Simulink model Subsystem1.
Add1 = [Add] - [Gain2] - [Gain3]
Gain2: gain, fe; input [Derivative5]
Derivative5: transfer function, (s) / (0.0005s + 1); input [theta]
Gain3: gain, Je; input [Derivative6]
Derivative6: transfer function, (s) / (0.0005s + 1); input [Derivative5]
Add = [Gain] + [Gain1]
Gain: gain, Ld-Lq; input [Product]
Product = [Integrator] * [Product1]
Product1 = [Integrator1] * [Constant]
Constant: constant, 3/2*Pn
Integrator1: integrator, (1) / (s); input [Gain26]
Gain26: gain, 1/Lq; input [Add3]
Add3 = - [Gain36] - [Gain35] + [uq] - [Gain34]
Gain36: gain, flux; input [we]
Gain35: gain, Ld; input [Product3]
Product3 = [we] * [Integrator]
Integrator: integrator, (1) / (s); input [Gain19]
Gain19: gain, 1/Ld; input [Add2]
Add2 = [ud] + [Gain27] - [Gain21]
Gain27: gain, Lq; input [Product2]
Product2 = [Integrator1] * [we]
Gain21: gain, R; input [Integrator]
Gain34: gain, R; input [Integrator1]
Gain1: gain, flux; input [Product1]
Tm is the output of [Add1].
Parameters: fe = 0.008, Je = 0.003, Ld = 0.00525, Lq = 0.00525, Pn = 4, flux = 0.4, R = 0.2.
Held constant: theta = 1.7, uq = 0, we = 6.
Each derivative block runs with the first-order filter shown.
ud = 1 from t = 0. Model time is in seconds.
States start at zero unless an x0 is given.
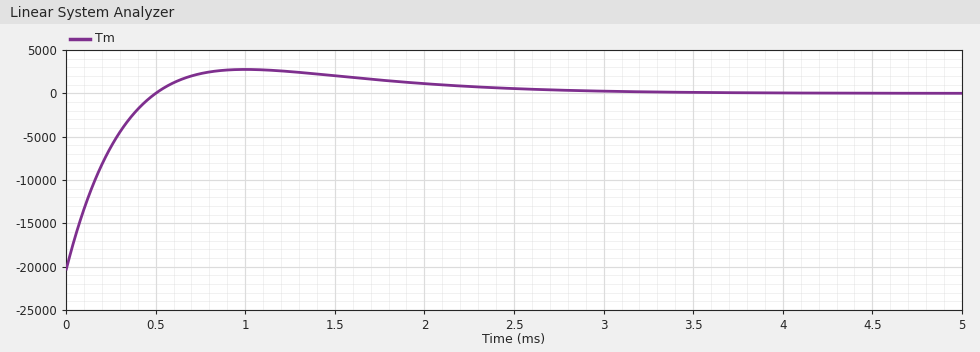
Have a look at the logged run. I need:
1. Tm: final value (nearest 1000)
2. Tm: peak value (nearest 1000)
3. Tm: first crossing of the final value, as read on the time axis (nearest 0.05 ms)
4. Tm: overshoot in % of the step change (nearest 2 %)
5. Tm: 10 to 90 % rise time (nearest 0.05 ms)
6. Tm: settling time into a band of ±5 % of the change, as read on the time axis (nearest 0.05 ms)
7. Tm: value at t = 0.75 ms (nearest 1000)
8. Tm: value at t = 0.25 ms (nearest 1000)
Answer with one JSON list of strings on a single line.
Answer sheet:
["0", "3000", "0.50 ms", "14 %", "0.35 ms", "2.10 ms", "2000", "-6000"]
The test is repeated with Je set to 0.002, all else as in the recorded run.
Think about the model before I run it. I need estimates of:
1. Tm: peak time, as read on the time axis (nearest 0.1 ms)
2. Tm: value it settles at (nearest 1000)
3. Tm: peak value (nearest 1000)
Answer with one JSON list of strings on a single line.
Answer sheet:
["1.0 ms", "0", "2000"]
